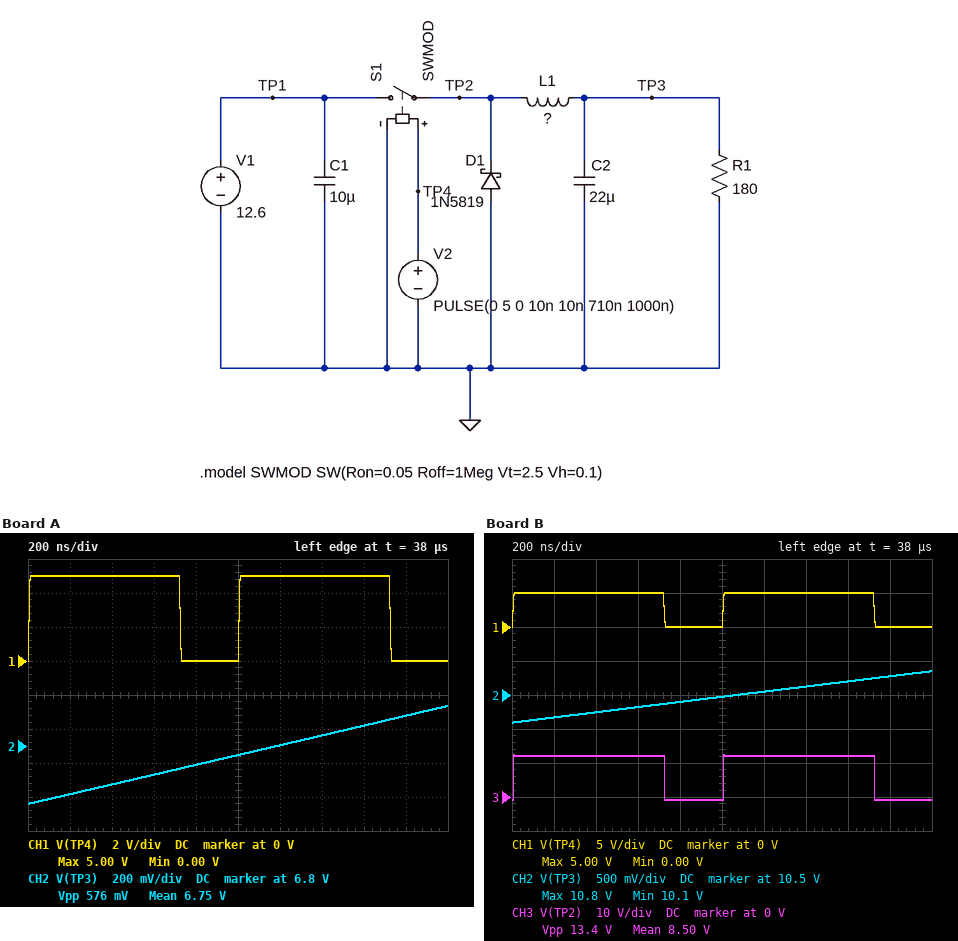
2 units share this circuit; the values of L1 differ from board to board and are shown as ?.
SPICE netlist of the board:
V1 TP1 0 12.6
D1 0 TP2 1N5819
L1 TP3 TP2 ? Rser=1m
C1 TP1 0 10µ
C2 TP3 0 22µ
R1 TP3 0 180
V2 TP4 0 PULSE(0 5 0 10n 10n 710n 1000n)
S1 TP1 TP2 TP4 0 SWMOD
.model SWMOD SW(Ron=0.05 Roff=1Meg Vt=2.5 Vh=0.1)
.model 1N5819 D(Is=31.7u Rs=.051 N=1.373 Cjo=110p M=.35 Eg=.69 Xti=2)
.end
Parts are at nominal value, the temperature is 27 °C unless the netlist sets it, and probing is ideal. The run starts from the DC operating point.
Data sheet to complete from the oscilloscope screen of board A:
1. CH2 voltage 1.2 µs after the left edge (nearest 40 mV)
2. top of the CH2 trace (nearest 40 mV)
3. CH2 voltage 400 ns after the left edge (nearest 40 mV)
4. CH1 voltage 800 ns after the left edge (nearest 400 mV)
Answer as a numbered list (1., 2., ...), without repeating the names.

1. 6.80 V
2. 7.04 V
3. 6.56 V
4. 0 V
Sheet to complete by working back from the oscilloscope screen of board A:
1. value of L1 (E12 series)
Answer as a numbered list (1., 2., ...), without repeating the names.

1. 39 µH
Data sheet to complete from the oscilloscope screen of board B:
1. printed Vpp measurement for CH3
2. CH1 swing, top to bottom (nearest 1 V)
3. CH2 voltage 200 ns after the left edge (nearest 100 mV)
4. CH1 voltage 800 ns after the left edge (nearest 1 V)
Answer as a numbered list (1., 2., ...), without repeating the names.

1. 13.4 V
2. 5 V
3. 10.2 V
4. 0 V
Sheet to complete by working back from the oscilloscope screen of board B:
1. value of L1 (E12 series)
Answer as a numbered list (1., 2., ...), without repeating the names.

1. 22 µH
